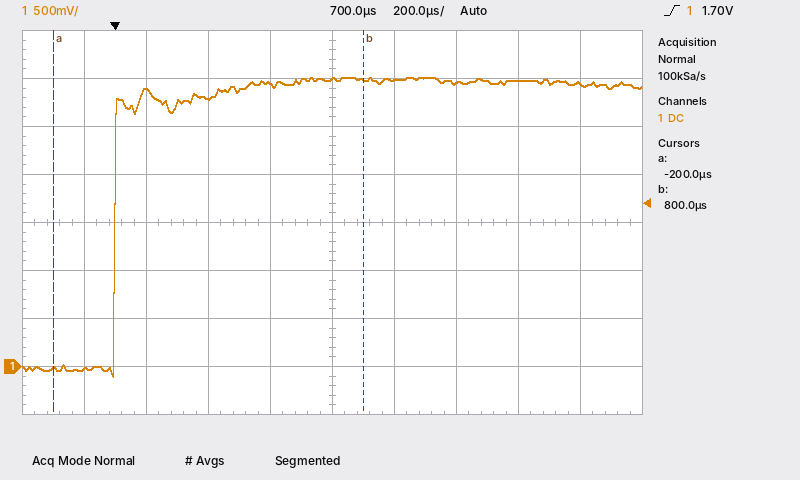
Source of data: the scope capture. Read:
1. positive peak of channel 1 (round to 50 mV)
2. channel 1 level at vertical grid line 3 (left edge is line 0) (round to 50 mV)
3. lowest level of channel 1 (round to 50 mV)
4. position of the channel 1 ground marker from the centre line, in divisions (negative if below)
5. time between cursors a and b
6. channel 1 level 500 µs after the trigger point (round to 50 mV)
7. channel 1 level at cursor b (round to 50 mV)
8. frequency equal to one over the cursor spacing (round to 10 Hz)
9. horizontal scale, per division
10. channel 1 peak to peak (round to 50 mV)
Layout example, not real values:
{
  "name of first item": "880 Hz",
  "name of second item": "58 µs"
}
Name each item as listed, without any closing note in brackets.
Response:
{
  "positive peak of channel 1": "3.00 V",
  "channel 1 level at vertical grid line 3 (left edge is line 0)": "2.80 V",
  "lowest level of channel 1": "-100 mV",
  "position of the channel 1 ground marker from the centre line, in divisions": "-3.0 div",
  "time between cursors a and b": "1.00 ms",
  "channel 1 level 500 µs after the trigger point": "2.95 V",
  "channel 1 level at cursor b": "3.00 V",
  "frequency equal to one over the cursor spacing": "1.00 kHz",
  "horizontal scale, per division": "200 µs",
  "channel 1 peak to peak": "3.10 V"
}
